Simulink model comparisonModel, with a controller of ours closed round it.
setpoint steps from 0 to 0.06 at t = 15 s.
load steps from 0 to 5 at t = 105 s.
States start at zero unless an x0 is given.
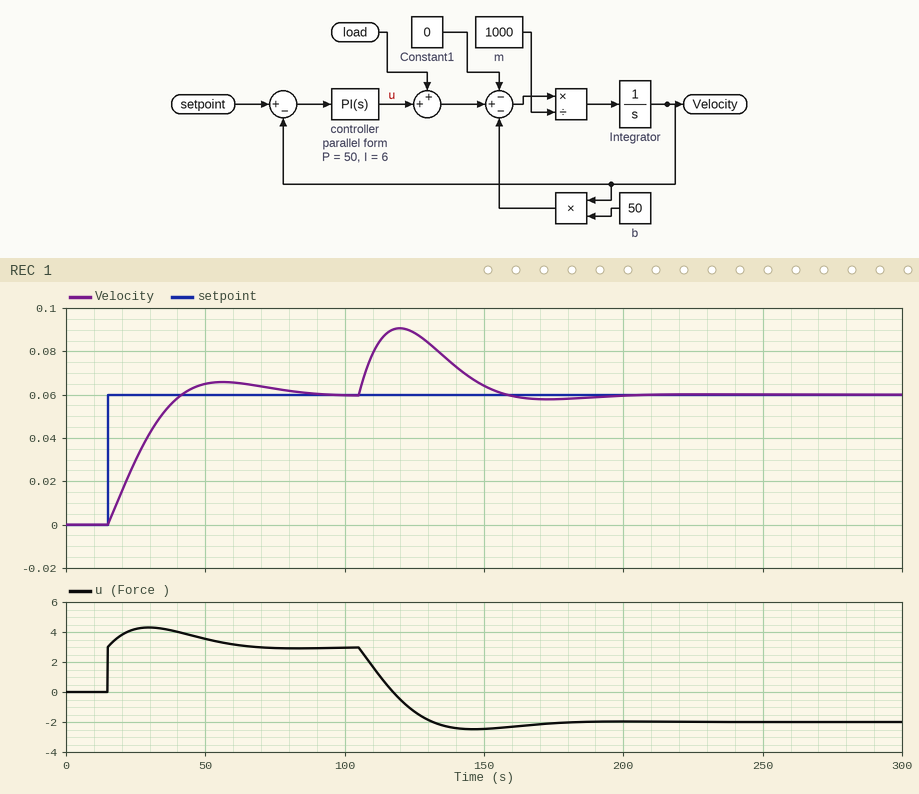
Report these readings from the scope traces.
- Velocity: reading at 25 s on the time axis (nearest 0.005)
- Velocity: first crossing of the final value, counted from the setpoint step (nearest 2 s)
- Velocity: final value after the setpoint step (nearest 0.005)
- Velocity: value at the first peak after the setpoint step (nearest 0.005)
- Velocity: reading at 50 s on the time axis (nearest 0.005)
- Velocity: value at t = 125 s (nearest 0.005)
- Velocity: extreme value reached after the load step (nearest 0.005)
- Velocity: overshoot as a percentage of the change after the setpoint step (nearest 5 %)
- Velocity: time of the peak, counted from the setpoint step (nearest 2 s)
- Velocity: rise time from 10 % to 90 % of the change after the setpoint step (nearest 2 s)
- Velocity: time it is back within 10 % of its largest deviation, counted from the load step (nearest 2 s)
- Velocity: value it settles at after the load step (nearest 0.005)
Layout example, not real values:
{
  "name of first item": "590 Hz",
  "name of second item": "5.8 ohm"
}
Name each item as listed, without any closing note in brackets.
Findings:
{
  "Velocity: reading at 25 s on the time axis": "0.030",
  "Velocity: first crossing of the final value, counted from the setpoint step": "26 s",
  "Velocity: final value after the setpoint step": "0.060",
  "Velocity: value at the first peak after the setpoint step": "0.065",
  "Velocity: reading at 50 s on the time axis": "0.065",
  "Velocity: value at t = 125 s": "0.090",
  "Velocity: extreme value reached after the load step": "0.090",
  "Velocity: overshoot as a percentage of the change after the setpoint step": "10 %",
  "Velocity: time of the peak, counted from the setpoint step": "42 s",
  "Velocity: rise time from 10 % to 90 % of the change after the setpoint step": "20 s",
  "Velocity: time it is back within 10 % of its largest deviation, counted from the load step": "46 s",
  "Velocity: value it settles at after the load step": "0.060"
}
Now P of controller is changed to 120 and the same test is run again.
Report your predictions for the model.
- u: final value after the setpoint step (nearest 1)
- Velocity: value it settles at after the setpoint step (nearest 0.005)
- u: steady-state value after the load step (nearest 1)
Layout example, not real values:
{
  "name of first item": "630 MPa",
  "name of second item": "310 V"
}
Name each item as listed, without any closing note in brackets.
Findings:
{
  "u: final value after the setpoint step": "3",
  "Velocity: value it settles at after the setpoint step": "0.060",
  "u: steady-state value after the load step": "-2"
}
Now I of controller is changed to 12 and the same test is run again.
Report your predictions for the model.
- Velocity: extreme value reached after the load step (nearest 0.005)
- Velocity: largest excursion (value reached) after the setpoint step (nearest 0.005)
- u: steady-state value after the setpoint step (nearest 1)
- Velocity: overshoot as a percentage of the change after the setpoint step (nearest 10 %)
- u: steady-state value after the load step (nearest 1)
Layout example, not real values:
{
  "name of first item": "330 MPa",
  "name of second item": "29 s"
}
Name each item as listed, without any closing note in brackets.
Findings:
{
  "Velocity: extreme value reached after the load step": "0.085",
  "Velocity: largest excursion (value reached) after the setpoint step": "0.075",
  "u: steady-state value after the setpoint step": "3",
  "Velocity: overshoot as a percentage of the change after the setpoint step": "20 %",
  "u: steady-state value after the load step": "-2"
}
